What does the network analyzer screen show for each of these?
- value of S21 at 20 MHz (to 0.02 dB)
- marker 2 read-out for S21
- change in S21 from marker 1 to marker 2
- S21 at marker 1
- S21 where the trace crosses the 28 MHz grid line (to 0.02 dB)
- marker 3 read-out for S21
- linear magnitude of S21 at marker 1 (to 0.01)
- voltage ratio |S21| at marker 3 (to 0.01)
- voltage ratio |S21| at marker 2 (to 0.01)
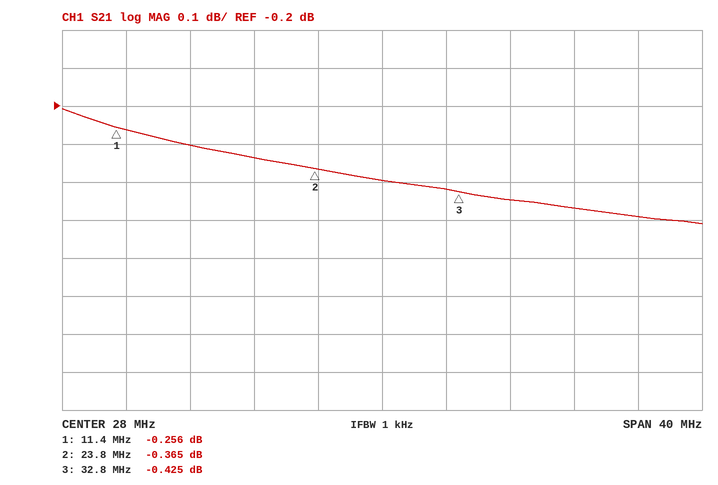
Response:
-0.34 dB
-0.365 dB
-0.109 dB
-0.256 dB
-0.40 dB
-0.425 dB
0.97
0.95
0.96
